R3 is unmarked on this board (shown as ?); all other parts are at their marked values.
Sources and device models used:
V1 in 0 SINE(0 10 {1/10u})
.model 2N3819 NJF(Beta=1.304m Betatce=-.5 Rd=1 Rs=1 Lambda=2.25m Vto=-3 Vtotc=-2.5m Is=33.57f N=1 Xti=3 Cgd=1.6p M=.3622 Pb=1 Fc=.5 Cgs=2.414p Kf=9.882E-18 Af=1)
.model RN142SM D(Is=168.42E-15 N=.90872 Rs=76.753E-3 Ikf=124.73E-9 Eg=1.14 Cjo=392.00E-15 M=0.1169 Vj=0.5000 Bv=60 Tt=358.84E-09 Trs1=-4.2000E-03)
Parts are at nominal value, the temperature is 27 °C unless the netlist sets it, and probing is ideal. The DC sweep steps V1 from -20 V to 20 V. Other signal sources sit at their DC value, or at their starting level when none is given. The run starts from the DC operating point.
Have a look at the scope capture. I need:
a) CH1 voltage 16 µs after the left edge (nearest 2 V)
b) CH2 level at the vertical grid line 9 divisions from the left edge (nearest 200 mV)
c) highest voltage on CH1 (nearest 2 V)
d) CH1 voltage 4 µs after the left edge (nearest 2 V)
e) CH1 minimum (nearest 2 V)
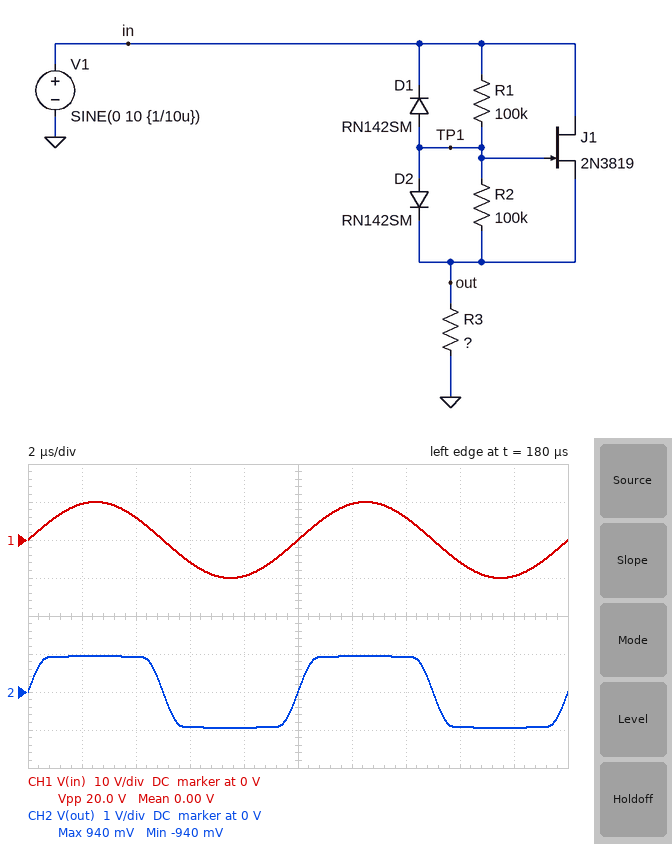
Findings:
-6 V
-1.0 V
10 V
6 V
-10 V
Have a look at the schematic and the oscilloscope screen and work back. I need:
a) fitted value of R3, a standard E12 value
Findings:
56 Ω
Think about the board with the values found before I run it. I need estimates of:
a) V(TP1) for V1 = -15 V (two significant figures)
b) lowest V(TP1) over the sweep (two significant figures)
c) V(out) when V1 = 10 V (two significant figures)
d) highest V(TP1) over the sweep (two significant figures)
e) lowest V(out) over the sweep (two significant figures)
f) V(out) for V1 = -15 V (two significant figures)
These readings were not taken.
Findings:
-14 V
-19 V
940 mV
1.6 V
-980 mV
-960 mV
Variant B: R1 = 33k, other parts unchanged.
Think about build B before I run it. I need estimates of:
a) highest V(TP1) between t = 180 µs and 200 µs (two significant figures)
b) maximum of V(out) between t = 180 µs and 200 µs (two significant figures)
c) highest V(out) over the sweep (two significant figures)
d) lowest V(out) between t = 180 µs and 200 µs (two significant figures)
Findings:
1.6 V
970 mV
1.0 V
-940 mV
